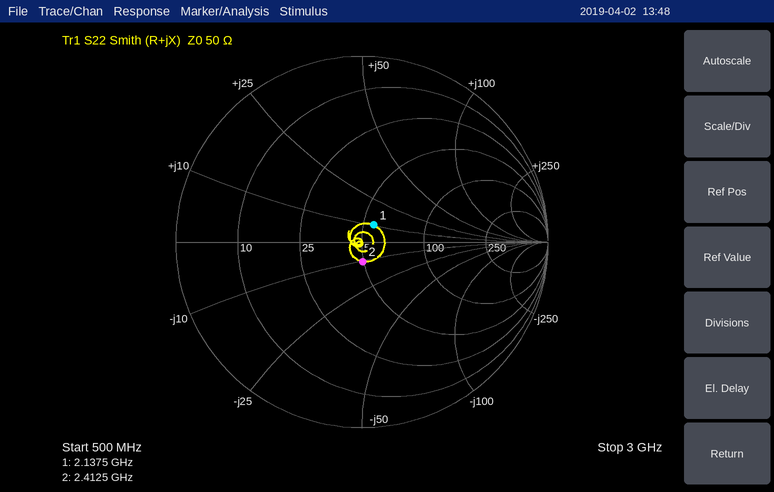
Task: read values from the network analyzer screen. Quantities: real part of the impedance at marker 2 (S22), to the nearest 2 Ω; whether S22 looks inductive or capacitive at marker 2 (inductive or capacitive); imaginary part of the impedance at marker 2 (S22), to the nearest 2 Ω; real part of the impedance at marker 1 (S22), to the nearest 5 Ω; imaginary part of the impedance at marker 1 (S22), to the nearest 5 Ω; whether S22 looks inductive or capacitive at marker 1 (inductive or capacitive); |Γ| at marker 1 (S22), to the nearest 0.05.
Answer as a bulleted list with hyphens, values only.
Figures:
- 50 Ω
- capacitive
- -10 Ω
- 55 Ω
- +10 Ω
- inductive
- 0.10
